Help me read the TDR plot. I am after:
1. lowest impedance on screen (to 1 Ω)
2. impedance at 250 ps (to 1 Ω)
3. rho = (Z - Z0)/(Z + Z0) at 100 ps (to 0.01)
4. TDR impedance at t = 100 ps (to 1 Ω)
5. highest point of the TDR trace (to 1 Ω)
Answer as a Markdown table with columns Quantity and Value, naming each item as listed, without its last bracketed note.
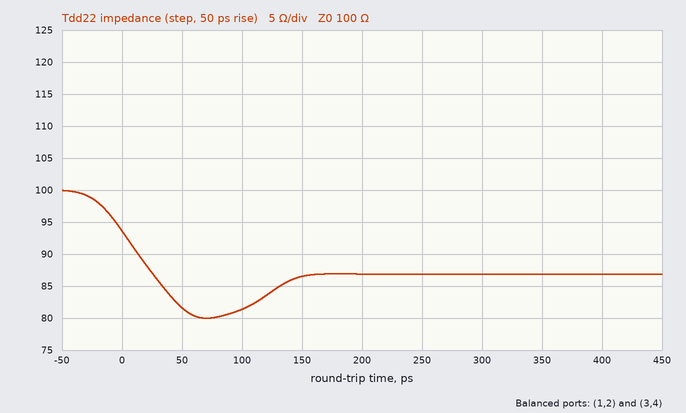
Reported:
| Quantity | Value |
|---|---|
| lowest impedance on screen | 80 Ω |
| impedance at 250 ps | 87 Ω |
| rho = (Z - Z0)/(Z + Z0) at 100 ps | -0.10 |
| TDR impedance at t = 100 ps | 81 Ω |
| highest point of the TDR trace | 100 Ω |
